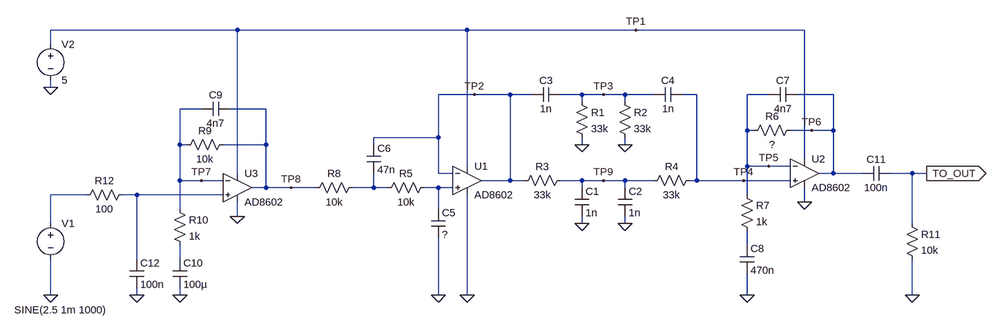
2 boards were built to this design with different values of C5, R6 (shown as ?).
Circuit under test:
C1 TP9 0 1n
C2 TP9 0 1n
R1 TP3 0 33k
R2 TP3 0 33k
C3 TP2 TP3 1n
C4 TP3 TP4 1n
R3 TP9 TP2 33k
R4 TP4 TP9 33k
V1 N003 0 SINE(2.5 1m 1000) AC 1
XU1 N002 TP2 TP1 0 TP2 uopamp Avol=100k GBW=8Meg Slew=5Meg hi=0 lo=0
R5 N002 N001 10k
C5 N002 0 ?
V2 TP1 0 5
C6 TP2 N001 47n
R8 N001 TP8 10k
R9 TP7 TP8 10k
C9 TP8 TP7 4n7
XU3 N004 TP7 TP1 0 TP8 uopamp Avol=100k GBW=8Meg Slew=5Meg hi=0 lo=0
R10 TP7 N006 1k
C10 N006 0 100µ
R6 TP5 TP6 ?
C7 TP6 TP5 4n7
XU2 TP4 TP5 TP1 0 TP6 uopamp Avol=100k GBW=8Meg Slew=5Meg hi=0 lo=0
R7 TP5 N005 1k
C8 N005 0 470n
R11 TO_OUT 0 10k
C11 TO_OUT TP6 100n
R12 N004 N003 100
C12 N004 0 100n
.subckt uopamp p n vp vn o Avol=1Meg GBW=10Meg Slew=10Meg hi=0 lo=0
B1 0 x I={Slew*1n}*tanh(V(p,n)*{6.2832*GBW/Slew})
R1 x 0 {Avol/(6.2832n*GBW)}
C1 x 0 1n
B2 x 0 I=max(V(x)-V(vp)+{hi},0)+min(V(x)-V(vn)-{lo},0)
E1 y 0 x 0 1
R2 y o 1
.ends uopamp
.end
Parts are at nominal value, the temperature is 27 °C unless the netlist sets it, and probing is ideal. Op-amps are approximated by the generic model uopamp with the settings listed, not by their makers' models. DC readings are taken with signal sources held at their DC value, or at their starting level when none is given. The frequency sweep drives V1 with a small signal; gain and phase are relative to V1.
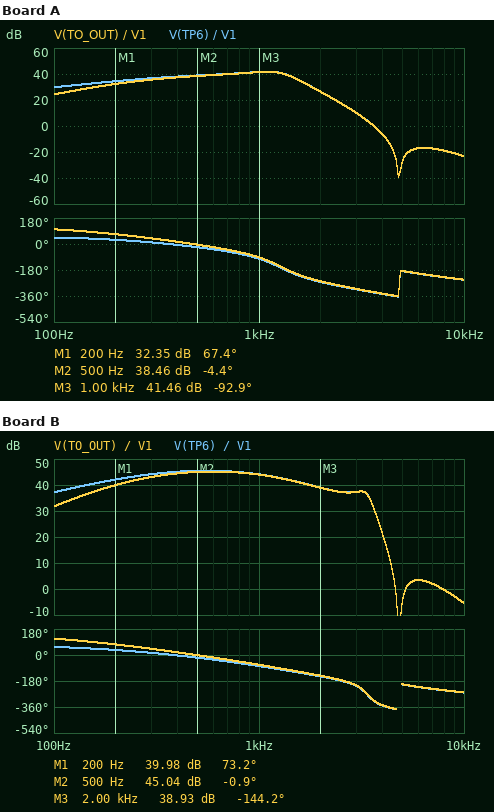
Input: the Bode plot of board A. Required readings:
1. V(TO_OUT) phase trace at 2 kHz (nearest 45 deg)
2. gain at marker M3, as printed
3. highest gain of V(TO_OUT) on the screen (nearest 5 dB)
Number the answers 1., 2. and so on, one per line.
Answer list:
1. -270 deg
2. 41.46 dB
3. 40 dB
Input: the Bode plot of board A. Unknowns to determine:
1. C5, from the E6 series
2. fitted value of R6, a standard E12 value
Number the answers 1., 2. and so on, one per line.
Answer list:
1. 3.3 nF
2. 8.2 kΩ
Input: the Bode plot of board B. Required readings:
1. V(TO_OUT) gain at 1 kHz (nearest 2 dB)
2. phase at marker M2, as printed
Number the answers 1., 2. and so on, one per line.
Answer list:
1. 44 dB
2. -0.9 deg
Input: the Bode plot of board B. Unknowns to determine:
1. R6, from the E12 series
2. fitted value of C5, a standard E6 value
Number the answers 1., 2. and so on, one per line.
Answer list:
1. 22 kΩ
2. 470 pF
